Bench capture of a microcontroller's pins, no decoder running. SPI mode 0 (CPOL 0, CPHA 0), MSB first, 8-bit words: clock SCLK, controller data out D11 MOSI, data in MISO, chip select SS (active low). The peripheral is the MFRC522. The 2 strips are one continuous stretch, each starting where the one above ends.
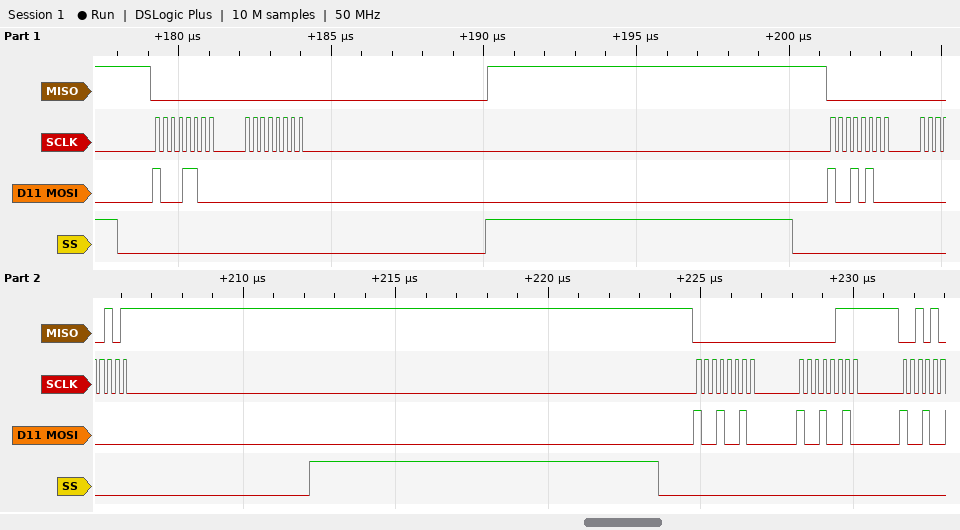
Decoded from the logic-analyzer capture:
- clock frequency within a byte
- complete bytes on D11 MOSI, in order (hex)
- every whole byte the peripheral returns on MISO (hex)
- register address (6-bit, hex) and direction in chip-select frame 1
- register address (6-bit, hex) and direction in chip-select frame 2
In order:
4 MHz
8C 00 94 00 92 92
00 00 00 05 00 07
0x06 read
0x0A read
